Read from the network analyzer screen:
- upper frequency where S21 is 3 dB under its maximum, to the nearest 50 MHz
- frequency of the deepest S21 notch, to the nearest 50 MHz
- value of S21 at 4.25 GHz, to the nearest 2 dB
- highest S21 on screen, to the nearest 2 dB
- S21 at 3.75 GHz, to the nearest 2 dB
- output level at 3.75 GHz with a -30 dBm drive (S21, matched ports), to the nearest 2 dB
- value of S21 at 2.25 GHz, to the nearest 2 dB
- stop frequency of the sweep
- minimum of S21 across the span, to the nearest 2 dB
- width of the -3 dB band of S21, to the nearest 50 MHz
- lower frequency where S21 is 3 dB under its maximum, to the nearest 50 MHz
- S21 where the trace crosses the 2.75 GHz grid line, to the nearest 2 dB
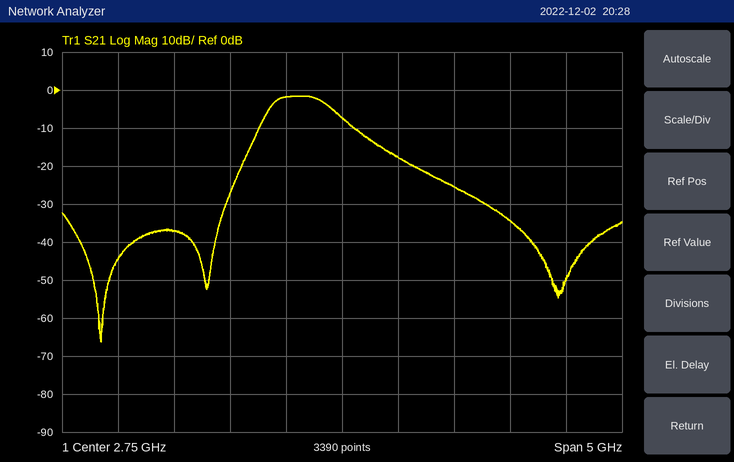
2.65 GHz
600 MHz
-34 dB
-2 dB
-26 dB
-56 dBm
-2 dB
5.25 GHz
-66 dB
550 MHz
2.10 GHz
-8 dB
